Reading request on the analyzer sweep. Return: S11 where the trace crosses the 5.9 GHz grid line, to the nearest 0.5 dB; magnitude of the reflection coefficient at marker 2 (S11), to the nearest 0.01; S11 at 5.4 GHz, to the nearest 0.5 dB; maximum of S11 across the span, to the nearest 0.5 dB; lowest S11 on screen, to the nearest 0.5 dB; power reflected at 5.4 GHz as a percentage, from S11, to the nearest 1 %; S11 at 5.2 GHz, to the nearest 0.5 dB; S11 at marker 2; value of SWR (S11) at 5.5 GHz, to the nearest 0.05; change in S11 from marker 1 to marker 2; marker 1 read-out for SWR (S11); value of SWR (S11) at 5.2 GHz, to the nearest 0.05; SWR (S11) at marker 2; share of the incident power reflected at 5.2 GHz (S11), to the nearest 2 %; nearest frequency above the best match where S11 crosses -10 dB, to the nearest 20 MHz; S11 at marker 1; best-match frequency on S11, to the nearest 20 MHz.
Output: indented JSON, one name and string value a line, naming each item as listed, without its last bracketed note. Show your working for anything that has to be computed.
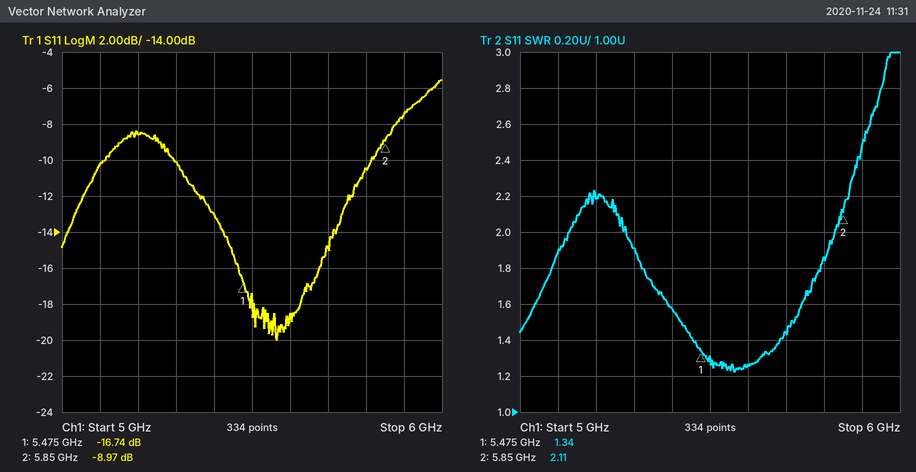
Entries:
{
  "S11 where the trace crosses the 5.9 GHz grid line, to the nearest 0.5 dB": "-7.5 dB",
  "magnitude of the reflection coefficient at marker 2 (S11), to the nearest 0.01": "10^(-8.97/20) ≈ 0.36",
  "S11 at 5.4 GHz, to the nearest 0.5 dB": "-13.0 dB",
  "maximum of S11 across the span, to the nearest 0.5 dB": "-5.5 dB",
  "lowest S11 on screen, to the nearest 0.5 dB": "-20.0 dB",
  "power reflected at 5.4 GHz as a percentage, from S11, to the nearest 1 %": "10^(-13/10) ≈ 5 %",
  "S11 at 5.2 GHz, to the nearest 0.5 dB": "-8.5 dB",
  "S11 at marker 2": "-8.97 dB",
  "value of SWR (S11) at 5.5 GHz, to the nearest 0.05": "1.30",
  "change in S11 from marker 1 to marker 2": "-8.97 − (-16.74) = 7.77 dB",
  "marker 1 read-out for SWR": "1.34",
  "value of SWR (S11) at 5.2 GHz, to the nearest 0.05": "2.20",
  "SWR (S11) at marker 2": "2.11",
  "share of the incident power reflected at 5.2 GHz (S11), to the nearest 2 %": "10^(-8.5/10) ≈ 14 %",
  "nearest frequency above the best match where S11 crosses -10 dB, to the nearest 20 MHz": "5.82 GHz",
  "S11 at marker 1": "-16.74 dB",
  "best-match frequency on S11, to the nearest 20 MHz": "5.56 GHz"
}
